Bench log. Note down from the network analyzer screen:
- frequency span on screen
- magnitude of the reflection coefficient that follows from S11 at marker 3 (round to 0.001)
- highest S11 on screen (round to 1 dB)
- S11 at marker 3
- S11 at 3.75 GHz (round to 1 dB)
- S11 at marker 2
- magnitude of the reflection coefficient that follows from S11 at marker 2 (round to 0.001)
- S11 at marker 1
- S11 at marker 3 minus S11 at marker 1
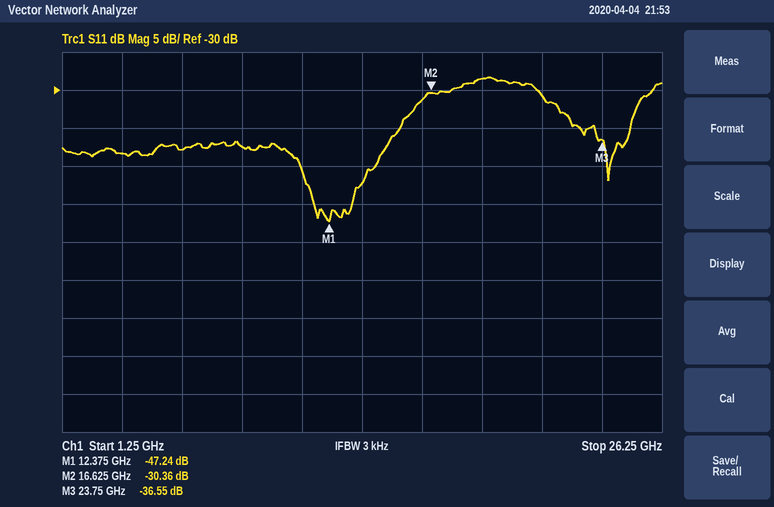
25 GHz
0.015
-28 dB
-36.55 dB
-38 dB
-30.36 dB
0.030
-47.24 dB
10.69 dB
